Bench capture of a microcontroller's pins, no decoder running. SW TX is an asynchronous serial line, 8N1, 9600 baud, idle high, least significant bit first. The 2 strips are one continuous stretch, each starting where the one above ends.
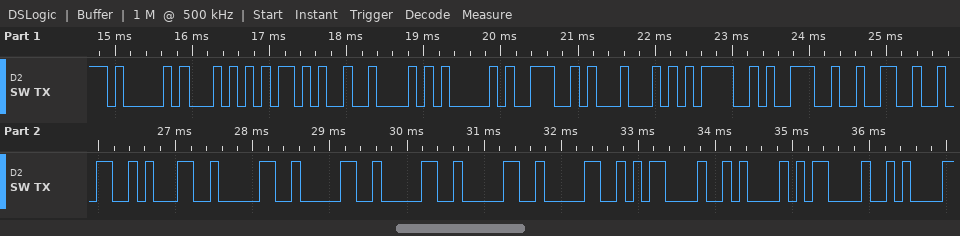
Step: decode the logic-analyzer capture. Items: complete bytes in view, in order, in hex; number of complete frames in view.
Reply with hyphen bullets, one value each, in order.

- 41 54 2B 42 41 4E 44 3D 39 32 32 31 30 30 30 30 30 0D 0A 0D 0A
- 21
